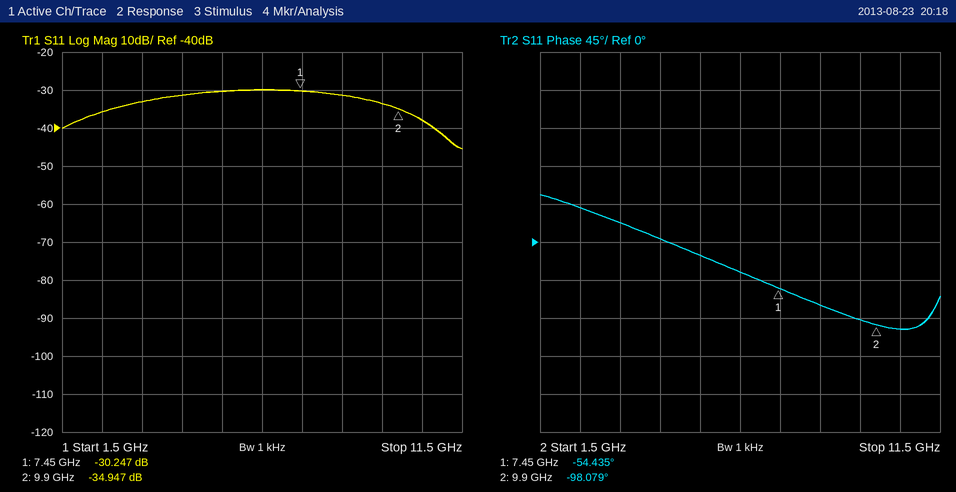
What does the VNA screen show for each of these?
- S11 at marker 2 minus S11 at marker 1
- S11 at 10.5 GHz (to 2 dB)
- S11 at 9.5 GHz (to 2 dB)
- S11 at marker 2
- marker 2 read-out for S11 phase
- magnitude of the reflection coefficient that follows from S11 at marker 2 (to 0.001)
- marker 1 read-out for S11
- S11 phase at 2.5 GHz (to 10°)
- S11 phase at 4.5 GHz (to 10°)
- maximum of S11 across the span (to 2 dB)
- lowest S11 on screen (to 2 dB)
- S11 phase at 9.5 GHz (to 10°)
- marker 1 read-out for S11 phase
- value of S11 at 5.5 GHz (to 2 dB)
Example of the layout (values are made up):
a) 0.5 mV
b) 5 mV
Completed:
a) -4.700 dB
b) -38 dB
c) -34 dB
d) -34.947 dB
e) -98.079°
f) 0.018
g) -30.247 dB
h) 40°
i) 0°
j) -30 dB
k) -46 dB
l) -90°
m) -54.435°
n) -30 dB
